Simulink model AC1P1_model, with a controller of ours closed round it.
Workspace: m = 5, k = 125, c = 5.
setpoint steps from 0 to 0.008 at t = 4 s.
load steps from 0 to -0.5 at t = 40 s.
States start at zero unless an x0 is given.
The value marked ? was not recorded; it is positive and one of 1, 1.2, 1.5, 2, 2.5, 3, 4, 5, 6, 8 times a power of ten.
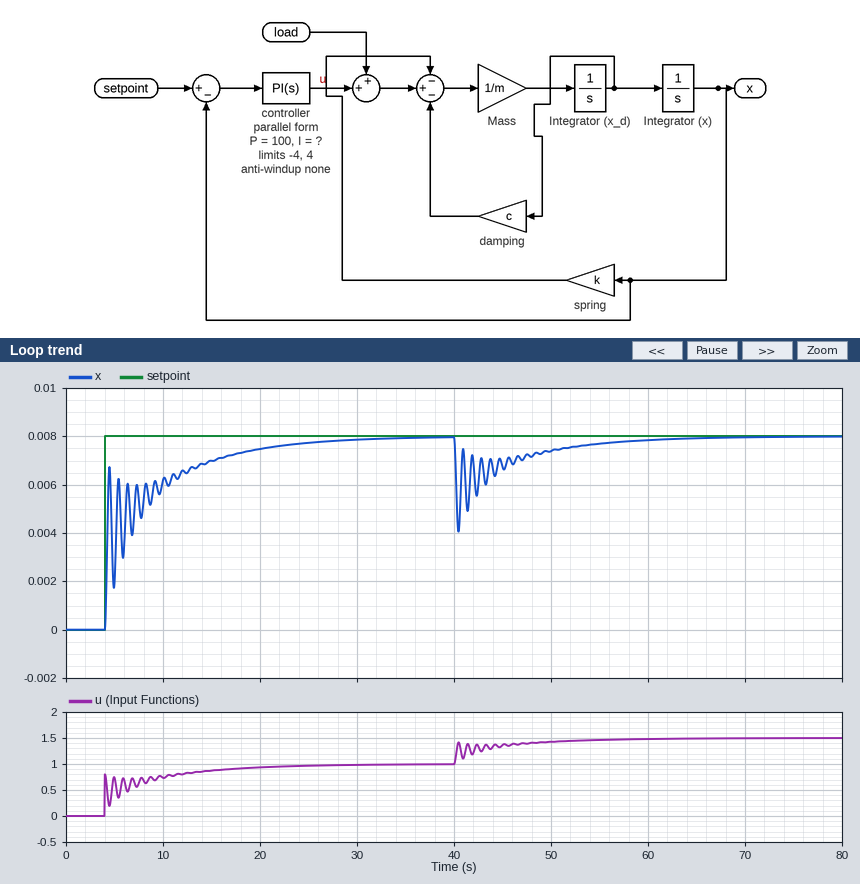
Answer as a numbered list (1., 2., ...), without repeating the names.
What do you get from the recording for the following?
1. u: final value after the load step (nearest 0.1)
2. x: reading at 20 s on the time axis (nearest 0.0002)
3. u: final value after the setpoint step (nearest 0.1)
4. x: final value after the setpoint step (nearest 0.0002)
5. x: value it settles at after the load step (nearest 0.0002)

1. 1.5
2. 0.0074
3. 1.0
4. 0.0080
5. 0.0080
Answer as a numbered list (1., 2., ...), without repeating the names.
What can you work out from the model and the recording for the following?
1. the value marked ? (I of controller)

1. 30
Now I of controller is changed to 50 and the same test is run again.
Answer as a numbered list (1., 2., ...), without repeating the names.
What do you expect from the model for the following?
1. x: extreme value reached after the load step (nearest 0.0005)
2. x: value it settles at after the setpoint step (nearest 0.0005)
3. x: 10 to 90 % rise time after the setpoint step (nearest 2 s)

1. 0.0040
2. 0.0080
3. 6 s
